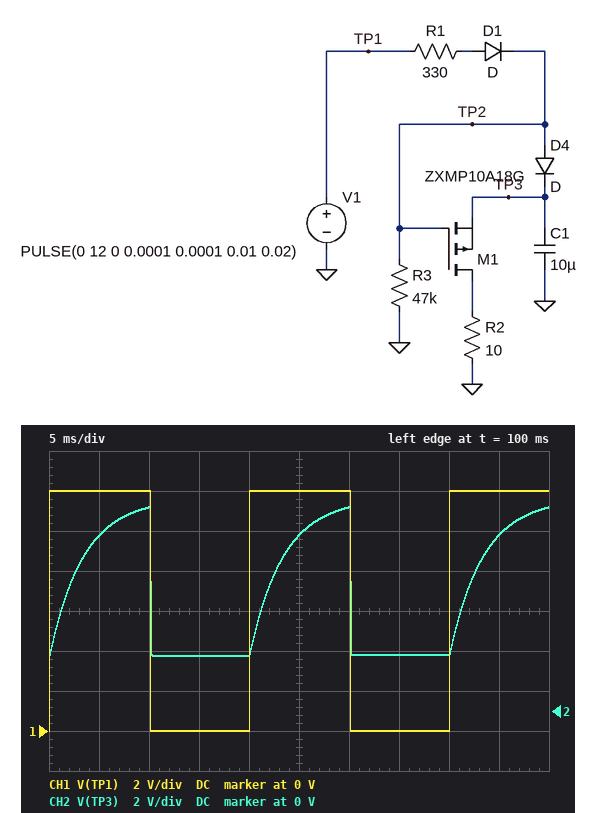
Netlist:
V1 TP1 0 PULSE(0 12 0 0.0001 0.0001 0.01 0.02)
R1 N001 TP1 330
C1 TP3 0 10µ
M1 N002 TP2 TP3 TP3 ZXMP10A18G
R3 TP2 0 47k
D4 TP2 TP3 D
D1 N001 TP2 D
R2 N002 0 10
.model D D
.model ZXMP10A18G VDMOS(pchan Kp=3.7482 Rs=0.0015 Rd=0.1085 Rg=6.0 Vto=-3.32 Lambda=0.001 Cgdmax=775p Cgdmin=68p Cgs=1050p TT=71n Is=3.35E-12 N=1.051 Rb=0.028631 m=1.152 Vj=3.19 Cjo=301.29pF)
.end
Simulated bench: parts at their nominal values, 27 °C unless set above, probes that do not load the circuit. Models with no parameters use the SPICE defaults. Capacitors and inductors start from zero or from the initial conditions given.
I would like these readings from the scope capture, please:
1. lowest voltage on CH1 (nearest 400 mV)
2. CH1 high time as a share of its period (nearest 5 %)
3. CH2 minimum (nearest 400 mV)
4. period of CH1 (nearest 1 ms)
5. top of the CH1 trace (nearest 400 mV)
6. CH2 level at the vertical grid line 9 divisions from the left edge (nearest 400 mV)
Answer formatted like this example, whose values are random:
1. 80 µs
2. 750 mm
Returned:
1. 0 V
2. 50 %
3. 2.8 V
4. 20 ms
5. 12.0 V
6. 8.8 V
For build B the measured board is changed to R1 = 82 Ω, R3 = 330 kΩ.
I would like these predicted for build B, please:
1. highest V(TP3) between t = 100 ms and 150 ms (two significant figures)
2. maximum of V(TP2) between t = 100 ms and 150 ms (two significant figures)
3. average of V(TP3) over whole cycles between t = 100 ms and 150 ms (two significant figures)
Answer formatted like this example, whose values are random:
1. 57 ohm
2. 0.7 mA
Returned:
1. 11 V
2. 11 V
3. 6.5 V
